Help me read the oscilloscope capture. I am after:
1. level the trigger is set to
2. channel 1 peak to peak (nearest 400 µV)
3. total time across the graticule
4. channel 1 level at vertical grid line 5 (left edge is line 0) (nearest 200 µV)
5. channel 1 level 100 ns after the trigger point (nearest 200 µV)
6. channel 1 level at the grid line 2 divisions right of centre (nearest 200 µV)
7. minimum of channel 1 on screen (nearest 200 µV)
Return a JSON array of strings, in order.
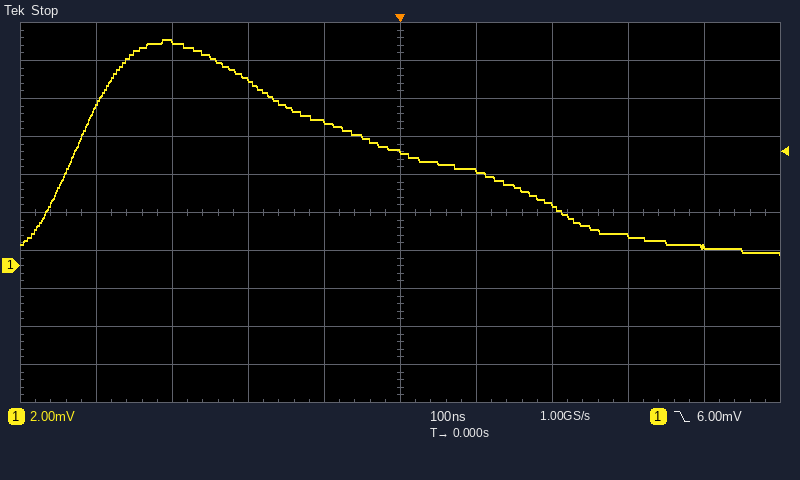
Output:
["6.00 mV", "11.2 mV", "1 µs", "6.0 mV", "5.0 mV", "3.2 mV", "600 µV"]
